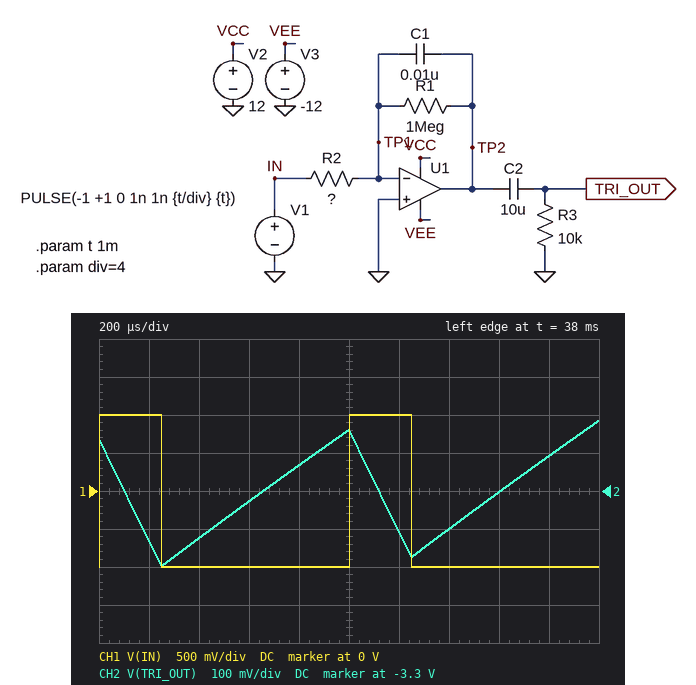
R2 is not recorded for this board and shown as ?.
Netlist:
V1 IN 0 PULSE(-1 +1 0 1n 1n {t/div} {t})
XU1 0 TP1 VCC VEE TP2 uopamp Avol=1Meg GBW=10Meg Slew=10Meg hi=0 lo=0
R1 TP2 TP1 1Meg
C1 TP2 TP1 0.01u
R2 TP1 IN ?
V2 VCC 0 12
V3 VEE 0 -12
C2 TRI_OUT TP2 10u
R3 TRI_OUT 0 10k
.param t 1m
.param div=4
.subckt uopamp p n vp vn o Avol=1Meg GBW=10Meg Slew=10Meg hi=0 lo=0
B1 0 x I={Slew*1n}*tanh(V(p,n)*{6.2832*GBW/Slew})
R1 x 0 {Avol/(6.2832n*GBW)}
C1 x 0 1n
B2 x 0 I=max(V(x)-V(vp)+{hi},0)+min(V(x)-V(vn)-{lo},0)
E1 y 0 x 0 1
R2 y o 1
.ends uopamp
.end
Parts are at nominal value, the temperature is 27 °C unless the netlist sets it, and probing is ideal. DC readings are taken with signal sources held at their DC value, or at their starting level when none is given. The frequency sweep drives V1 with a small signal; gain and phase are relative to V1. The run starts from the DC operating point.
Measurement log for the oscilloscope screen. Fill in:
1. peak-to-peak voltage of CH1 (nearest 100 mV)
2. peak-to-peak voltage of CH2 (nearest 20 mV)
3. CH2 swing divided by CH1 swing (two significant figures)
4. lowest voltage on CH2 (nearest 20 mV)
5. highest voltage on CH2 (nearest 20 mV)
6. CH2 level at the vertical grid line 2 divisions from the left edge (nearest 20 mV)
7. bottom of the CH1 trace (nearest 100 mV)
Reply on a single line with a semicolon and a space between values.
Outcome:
2.0 V; 380 mV; 0.19; -3.50 V; -3.12 V; -3.42 V; -1.0 V
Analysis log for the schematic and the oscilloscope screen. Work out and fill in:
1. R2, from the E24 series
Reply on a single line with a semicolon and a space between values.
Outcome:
110 kΩ
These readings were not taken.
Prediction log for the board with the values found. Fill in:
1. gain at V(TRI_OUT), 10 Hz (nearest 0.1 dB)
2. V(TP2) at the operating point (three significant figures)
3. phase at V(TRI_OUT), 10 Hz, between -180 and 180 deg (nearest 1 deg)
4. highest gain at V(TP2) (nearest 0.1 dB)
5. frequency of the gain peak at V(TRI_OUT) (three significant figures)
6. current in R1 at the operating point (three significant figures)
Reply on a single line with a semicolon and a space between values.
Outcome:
17.6 dB; 9.09 V; 157 deg; 19.2 dB; 5.03 Hz; 9.09 µA
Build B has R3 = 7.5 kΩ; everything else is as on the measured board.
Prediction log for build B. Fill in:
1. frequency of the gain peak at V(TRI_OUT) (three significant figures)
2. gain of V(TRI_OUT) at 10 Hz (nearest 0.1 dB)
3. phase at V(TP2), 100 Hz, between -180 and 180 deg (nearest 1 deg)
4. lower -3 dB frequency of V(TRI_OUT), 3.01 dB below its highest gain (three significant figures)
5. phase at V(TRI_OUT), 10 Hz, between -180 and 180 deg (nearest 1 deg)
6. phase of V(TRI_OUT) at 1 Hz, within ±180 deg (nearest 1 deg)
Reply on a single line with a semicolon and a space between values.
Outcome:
5.81 Hz; 17.5 dB; 99 deg; 1.71 Hz; 160 deg; -119 deg
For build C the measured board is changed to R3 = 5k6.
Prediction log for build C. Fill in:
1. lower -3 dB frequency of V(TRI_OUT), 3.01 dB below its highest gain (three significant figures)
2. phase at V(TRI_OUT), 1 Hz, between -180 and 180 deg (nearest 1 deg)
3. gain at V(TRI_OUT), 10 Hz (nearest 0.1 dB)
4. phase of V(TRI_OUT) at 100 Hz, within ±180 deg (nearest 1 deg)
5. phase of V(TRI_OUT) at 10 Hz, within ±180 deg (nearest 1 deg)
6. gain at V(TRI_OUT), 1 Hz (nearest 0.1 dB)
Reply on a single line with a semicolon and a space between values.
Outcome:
2.16 Hz; -113 deg; 17.4 dB; 101 deg; 164 deg; 9.6 dB
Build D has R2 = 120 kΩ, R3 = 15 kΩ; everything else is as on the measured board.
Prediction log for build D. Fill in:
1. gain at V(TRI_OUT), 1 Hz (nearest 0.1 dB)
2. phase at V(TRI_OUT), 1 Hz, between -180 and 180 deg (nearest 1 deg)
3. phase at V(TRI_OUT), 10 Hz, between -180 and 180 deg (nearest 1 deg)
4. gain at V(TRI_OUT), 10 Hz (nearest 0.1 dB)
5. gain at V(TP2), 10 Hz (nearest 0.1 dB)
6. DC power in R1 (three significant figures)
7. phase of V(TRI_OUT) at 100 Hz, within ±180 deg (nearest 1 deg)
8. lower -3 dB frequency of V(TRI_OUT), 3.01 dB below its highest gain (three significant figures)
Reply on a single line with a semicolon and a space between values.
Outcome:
15.1 dB; -137 deg; 154 deg; 16.9 dB; 17.0 dB; 69.4 µW; 100 deg; 942 mHz
